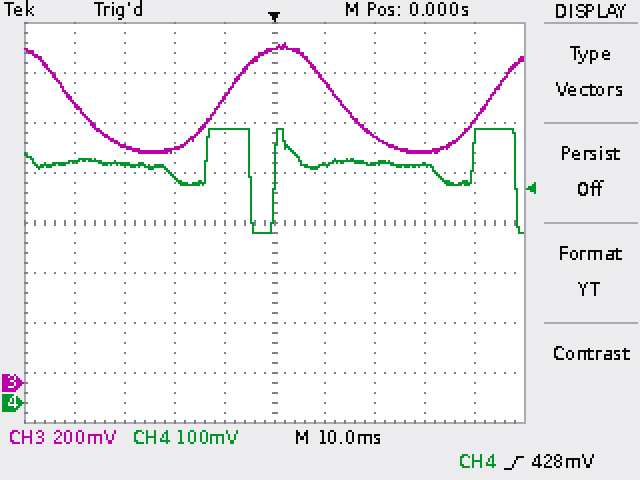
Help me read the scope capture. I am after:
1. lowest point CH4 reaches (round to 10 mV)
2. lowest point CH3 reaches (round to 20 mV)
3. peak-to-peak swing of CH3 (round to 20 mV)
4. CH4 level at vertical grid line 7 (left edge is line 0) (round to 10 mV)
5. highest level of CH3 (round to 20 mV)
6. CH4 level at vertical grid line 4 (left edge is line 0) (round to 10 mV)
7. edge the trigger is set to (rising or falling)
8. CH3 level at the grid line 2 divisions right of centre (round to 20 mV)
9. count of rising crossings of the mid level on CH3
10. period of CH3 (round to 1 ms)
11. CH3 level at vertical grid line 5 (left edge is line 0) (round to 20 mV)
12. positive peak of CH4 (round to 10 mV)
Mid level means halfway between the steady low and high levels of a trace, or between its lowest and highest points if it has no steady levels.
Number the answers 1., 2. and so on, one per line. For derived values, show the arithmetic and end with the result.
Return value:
1. 340 mV
2. 920 mV
3. 1.36 V − (920 mV) = 440 mV
4. 480 mV
5. 1.36 V
6. 550 mV
7. rising
8. 980 mV
9. 2
10. 53 ms
11. 1.34 V
12. 550 mV
